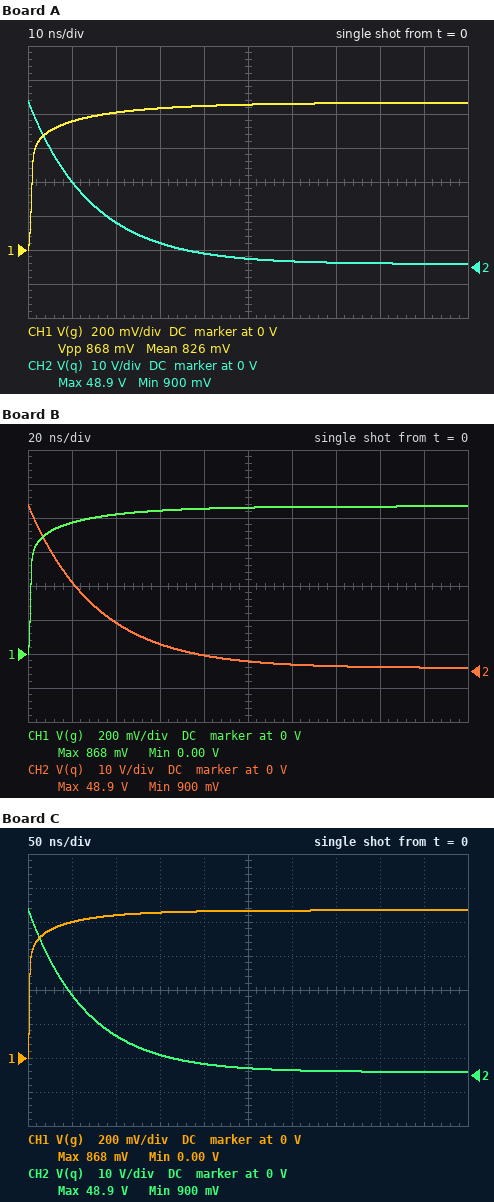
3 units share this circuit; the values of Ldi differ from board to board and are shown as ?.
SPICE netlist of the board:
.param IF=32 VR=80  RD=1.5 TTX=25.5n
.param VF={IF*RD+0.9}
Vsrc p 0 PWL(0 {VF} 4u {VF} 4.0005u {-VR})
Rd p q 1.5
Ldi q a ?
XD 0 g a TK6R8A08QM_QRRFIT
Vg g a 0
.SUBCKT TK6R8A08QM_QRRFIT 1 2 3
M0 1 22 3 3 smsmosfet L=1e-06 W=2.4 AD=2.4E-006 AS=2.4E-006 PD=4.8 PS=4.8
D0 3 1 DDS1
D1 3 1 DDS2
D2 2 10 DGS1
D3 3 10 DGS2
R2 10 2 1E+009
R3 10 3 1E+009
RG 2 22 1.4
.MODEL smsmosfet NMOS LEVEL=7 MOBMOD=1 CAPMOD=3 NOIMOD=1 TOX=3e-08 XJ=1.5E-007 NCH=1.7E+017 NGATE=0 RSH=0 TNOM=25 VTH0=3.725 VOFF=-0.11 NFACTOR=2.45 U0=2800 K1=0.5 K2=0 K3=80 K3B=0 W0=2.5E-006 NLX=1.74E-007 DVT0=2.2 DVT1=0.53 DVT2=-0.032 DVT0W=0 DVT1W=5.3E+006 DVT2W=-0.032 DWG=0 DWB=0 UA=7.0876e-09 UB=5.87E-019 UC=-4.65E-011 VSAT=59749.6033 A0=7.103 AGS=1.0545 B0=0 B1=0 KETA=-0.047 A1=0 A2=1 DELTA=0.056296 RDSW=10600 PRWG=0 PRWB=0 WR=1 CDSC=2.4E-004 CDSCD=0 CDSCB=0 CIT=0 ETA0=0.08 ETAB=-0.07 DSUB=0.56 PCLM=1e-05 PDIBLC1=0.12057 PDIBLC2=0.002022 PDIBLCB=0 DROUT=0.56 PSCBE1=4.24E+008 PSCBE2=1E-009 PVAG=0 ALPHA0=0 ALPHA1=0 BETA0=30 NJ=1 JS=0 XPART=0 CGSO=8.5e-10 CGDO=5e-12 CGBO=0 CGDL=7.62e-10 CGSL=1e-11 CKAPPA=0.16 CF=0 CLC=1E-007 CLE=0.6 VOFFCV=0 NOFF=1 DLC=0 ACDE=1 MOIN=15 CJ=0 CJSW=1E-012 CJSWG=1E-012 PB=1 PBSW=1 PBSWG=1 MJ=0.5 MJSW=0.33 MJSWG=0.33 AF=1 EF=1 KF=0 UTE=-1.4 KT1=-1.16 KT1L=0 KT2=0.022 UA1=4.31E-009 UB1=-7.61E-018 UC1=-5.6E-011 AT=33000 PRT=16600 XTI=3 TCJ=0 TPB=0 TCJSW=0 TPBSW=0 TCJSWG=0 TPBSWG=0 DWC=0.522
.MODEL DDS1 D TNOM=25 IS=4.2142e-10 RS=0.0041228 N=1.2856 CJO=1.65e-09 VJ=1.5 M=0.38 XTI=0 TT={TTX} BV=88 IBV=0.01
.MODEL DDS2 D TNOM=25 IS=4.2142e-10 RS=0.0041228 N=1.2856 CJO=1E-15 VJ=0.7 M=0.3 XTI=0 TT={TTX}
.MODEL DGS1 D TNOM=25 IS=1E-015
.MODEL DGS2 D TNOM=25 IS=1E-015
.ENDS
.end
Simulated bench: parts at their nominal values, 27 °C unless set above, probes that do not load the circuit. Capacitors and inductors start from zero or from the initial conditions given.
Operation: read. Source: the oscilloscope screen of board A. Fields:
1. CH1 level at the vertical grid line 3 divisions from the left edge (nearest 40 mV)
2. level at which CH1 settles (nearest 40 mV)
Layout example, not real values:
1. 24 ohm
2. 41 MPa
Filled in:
1. 840 mV
2. 880 mV
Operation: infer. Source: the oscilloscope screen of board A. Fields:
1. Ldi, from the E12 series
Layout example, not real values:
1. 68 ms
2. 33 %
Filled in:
1. 22 nH
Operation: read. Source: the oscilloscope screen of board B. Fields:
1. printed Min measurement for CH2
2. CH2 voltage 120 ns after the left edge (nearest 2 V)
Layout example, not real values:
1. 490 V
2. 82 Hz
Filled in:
1. 900 mV
2. 2 V
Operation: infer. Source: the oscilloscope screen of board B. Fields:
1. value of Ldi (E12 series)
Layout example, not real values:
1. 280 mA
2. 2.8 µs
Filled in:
1. 47 nH
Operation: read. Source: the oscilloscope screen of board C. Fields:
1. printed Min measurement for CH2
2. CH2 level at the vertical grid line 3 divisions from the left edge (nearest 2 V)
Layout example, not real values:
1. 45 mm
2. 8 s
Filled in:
1. 900 mV
2. 6 V
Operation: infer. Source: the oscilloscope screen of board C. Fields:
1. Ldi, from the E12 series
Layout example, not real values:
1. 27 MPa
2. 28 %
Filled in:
1. 100 nH
